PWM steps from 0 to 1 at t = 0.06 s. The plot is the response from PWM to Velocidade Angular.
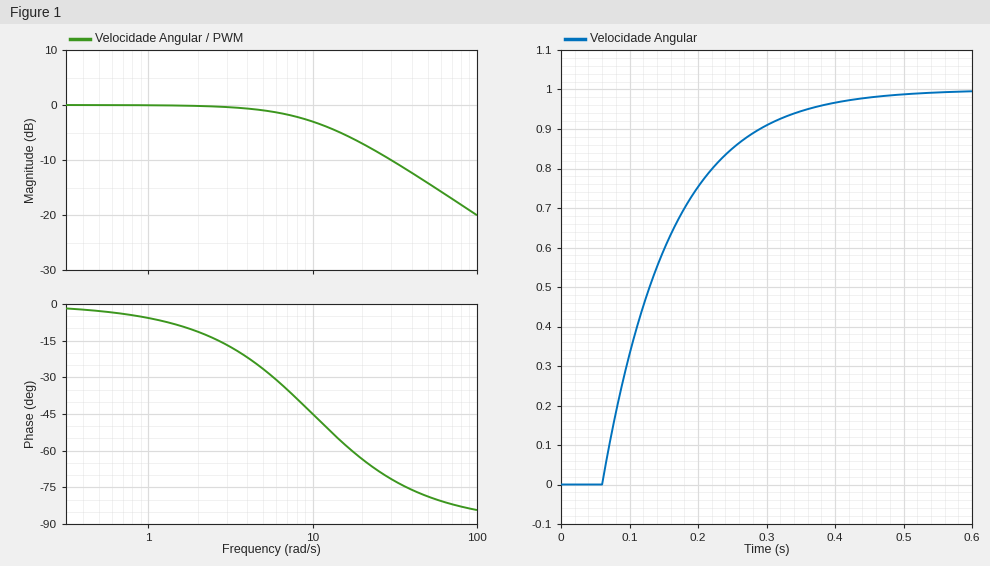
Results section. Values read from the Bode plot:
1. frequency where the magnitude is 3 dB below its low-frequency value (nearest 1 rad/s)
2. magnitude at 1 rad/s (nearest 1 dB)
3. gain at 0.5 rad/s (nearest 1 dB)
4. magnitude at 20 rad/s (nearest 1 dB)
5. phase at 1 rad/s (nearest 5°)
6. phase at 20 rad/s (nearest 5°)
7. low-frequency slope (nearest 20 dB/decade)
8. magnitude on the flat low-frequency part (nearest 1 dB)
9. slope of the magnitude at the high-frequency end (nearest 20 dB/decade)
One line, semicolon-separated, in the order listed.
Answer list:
10 rad/s; 0 dB; 0 dB; -7 dB; -5°; -65°; 0 dB/decade; 0 dB; -20 dB/decade
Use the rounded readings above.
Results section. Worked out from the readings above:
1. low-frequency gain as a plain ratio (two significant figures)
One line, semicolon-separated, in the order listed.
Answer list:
1.0
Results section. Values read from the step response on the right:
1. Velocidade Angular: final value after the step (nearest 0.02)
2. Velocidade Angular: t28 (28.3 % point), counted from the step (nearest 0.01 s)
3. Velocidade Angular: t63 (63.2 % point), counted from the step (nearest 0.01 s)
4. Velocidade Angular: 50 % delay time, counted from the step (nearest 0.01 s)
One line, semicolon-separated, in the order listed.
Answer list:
1.00; 0.03 s; 0.10 s; 0.07 s
